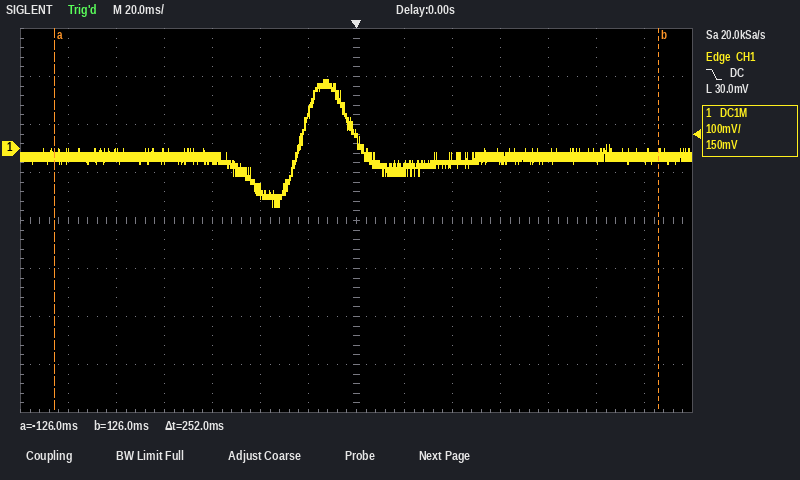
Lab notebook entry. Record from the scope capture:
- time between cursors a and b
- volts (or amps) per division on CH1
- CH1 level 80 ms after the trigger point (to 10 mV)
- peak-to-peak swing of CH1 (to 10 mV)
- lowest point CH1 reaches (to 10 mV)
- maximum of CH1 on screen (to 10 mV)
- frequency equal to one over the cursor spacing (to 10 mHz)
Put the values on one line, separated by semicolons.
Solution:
252 ms; 100 mV; -20 mV; 260 mV; -120 mV; 140 mV; 3.97 Hz
